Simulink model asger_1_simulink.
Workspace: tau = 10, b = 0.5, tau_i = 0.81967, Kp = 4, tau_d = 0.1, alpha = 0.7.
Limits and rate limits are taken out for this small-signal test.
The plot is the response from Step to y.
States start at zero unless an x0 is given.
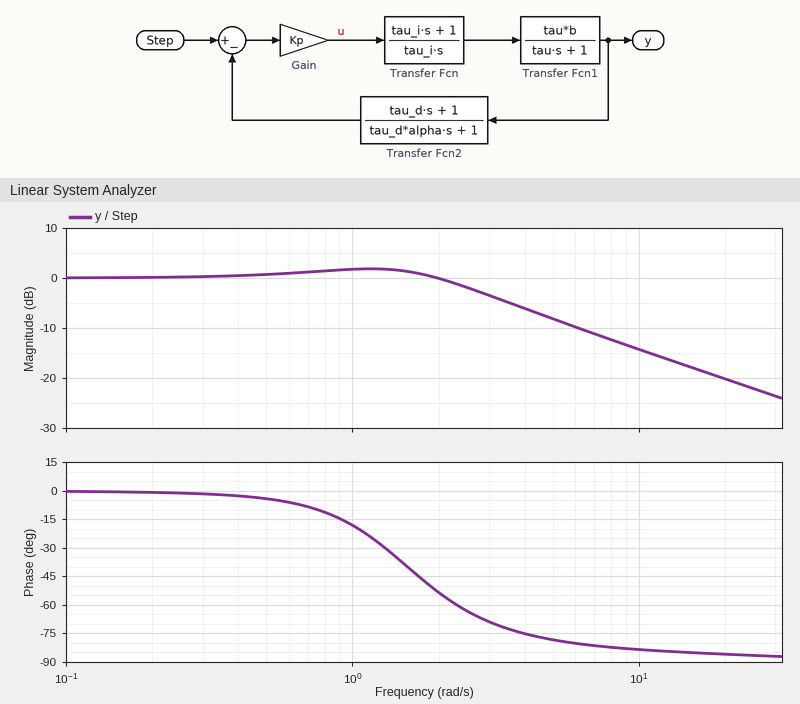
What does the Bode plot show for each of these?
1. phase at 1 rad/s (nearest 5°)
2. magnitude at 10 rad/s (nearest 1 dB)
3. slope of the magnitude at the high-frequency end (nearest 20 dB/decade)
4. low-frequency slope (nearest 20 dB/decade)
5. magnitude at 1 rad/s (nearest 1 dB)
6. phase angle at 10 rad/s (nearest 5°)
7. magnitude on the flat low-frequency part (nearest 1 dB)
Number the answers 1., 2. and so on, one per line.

1. -20°
2. -14 dB
3. -20 dB/decade
4. 0 dB/decade
5. 2 dB
6. -85°
7. 0 dB
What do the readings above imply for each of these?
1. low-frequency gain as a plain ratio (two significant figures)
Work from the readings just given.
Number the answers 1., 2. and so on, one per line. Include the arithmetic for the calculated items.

1. 10^(0 / 20) = 1.0
